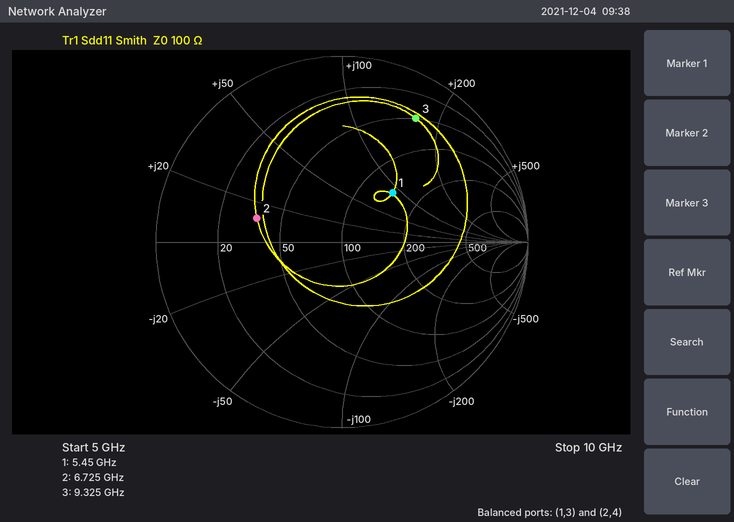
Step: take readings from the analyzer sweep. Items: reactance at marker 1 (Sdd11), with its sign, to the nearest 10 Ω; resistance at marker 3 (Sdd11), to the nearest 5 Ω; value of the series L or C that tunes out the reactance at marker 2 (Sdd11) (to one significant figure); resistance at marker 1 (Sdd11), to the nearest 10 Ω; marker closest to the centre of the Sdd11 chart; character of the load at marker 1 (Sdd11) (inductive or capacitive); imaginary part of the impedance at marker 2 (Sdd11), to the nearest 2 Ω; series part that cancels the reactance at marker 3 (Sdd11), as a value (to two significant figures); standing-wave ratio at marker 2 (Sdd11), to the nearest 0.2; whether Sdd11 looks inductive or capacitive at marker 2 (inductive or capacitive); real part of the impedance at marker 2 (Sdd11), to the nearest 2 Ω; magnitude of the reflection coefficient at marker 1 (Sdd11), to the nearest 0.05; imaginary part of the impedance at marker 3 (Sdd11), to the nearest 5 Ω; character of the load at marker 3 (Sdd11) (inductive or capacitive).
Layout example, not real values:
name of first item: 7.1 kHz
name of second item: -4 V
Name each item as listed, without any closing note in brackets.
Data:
reactance at marker 1 (Sdd11), with its sign, to the nearest 10 Ω: +90 Ω
resistance at marker 3 (Sdd11), to the nearest 5 Ω: 50 Ω
value of the series L or C that tunes out the reactance at marker 2 (Sdd11): 2 pF
resistance at marker 1 (Sdd11), to the nearest 10 Ω: 140 Ω
marker closest to the centre of the Sdd11 chart: marker 1
character of the load at marker 1 (Sdd11): inductive
imaginary part of the impedance at marker 2 (Sdd11), to the nearest 2 Ω: +12 Ω
series part that cancels the reactance at marker 3 (Sdd11), as a value: 100 fF
standing-wave ratio at marker 2 (Sdd11), to the nearest 0.2: 2.8
whether Sdd11 looks inductive or capacitive at marker 2: inductive
real part of the impedance at marker 2 (Sdd11), to the nearest 2 Ω: 36 Ω
magnitude of the reflection coefficient at marker 1 (Sdd11), to the nearest 0.05: 0.40
imaginary part of the impedance at marker 3 (Sdd11), to the nearest 5 Ω: +165 Ω
character of the load at marker 3 (Sdd11): inductive
